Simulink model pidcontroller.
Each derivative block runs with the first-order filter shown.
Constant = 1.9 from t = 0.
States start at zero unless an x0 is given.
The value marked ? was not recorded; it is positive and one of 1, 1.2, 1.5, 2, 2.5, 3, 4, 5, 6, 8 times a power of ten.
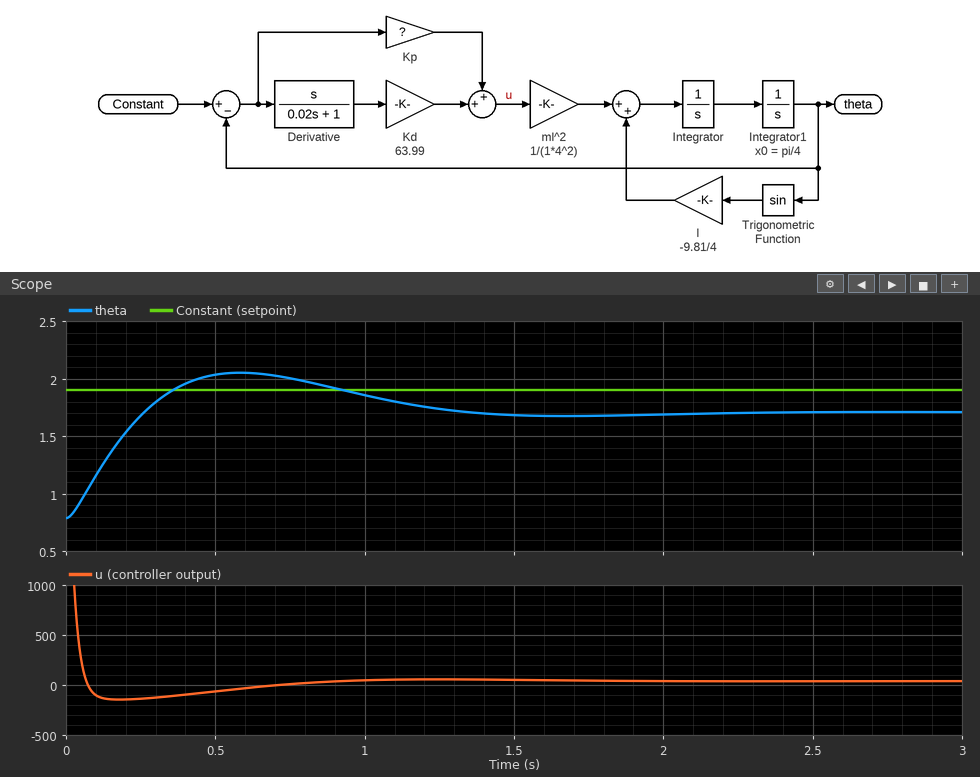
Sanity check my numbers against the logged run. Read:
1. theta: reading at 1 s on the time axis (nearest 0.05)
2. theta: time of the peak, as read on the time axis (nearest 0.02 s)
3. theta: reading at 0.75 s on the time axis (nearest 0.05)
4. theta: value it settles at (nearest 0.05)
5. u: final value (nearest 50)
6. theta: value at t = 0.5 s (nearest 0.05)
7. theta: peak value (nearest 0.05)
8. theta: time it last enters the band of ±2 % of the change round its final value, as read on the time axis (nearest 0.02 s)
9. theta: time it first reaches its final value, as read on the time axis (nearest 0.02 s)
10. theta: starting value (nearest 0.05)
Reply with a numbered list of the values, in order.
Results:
1. 1.85
2. 0.58 s
3. 2.00
4. 1.70
5. 50
6. 2.05
7. 2.05
8. 2.00 s
9. 0.26 s
10. 0.80
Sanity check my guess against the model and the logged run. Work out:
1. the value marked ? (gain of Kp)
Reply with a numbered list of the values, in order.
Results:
1. 200
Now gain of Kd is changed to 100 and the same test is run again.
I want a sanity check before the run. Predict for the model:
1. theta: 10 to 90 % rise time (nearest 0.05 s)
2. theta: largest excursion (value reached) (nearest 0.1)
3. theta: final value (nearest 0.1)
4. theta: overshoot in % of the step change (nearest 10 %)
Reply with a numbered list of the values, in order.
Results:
1. 0.15 s
2. 2.0
3. 1.7
4. 30 %
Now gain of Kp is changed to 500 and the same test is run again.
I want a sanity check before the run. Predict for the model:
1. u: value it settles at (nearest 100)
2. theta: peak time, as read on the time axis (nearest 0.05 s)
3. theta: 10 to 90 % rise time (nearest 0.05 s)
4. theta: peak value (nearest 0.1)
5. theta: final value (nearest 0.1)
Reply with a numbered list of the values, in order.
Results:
1. 0
2. 0.45 s
3. 0.15 s
4. 2.3
5. 1.8
